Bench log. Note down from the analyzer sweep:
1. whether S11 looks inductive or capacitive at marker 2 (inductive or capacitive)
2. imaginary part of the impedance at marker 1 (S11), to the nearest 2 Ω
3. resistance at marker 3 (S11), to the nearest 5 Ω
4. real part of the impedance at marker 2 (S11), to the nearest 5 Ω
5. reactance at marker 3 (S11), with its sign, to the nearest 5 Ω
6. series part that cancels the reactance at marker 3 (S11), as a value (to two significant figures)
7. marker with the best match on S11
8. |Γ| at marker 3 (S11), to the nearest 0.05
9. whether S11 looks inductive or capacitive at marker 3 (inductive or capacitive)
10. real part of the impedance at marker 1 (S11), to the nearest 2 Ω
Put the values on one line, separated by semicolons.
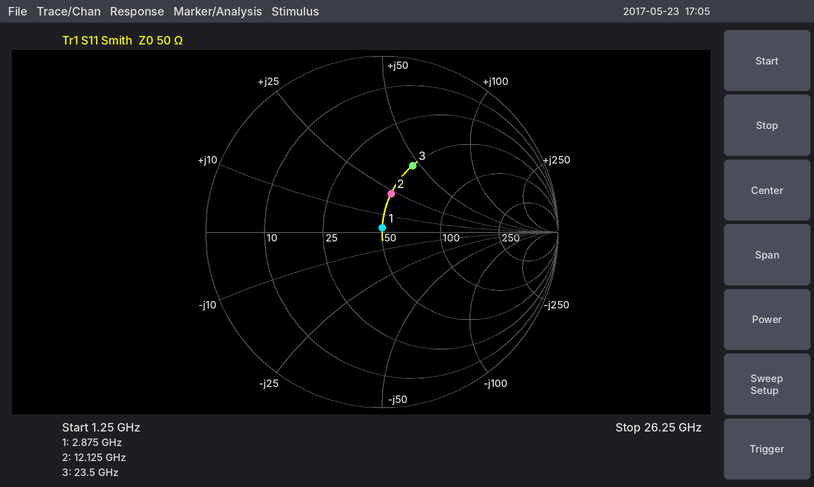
inductive; +2 Ω; 50 Ω; 50 Ω; +45 Ω; 150 fF; marker 1; 0.40; inductive; 50 Ω
